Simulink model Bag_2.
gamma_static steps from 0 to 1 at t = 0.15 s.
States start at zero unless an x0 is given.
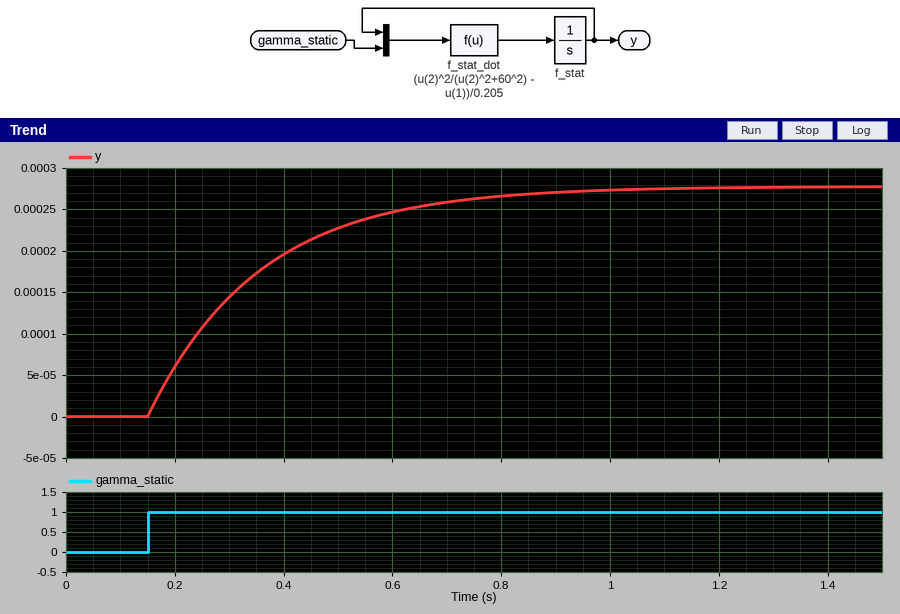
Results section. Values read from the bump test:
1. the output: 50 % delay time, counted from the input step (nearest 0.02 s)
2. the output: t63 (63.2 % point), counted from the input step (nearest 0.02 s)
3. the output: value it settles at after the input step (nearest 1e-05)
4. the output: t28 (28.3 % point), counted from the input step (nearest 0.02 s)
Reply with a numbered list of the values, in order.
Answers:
1. 0.14 s
2. 0.20 s
3. 0.00028
4. 0.06 s
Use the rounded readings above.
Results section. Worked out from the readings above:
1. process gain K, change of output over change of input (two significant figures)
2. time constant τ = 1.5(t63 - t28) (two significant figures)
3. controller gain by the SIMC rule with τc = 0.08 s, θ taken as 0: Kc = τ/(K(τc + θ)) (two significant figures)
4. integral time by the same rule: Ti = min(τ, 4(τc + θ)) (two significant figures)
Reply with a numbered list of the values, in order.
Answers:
1. 0.00028
2. 0.21 s
3. 9400
4. 0.21 s
